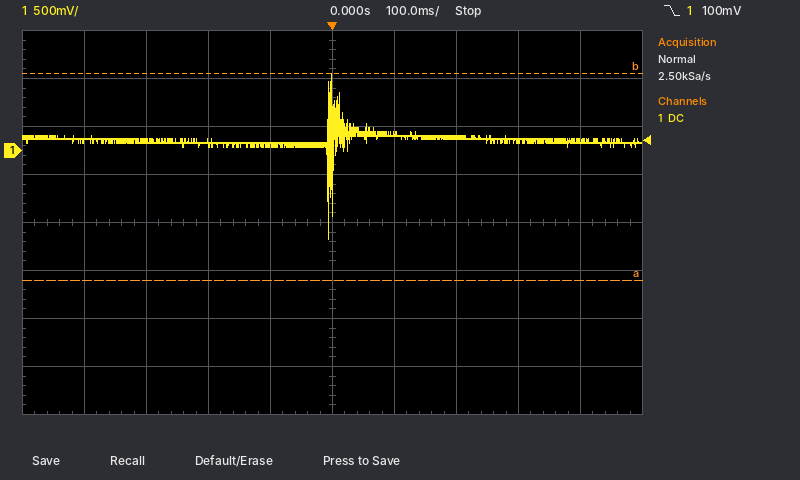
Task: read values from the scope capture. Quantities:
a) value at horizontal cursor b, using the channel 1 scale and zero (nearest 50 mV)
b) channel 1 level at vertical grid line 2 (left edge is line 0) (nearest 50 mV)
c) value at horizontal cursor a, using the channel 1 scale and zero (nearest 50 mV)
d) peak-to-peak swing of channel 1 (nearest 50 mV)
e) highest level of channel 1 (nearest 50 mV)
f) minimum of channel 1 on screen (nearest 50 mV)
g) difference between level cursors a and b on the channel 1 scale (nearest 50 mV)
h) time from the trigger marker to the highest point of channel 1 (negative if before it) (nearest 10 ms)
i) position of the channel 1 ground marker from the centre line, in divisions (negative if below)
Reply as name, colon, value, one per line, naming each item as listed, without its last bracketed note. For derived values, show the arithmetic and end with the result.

value at horizontal cursor b, using the channel 1 scale and zero: 800 mV
channel 1 level at vertical grid line 2 (left edge is line 0): 100 mV
value at horizontal cursor a, using the channel 1 scale and zero: -1.35 V
peak-to-peak swing of channel 1: 800 mV − (-900 mV) = 1.70 V
highest level of channel 1: 800 mV
minimum of channel 1 on screen: -900 mV
difference between level cursors a and b on the channel 1 scale: 2.15 V
time from the trigger marker to the highest point of channel 1 (negative if before it): 0 ms
position of the channel 1 ground marker from the centre line, in divisions: +1.5 div
